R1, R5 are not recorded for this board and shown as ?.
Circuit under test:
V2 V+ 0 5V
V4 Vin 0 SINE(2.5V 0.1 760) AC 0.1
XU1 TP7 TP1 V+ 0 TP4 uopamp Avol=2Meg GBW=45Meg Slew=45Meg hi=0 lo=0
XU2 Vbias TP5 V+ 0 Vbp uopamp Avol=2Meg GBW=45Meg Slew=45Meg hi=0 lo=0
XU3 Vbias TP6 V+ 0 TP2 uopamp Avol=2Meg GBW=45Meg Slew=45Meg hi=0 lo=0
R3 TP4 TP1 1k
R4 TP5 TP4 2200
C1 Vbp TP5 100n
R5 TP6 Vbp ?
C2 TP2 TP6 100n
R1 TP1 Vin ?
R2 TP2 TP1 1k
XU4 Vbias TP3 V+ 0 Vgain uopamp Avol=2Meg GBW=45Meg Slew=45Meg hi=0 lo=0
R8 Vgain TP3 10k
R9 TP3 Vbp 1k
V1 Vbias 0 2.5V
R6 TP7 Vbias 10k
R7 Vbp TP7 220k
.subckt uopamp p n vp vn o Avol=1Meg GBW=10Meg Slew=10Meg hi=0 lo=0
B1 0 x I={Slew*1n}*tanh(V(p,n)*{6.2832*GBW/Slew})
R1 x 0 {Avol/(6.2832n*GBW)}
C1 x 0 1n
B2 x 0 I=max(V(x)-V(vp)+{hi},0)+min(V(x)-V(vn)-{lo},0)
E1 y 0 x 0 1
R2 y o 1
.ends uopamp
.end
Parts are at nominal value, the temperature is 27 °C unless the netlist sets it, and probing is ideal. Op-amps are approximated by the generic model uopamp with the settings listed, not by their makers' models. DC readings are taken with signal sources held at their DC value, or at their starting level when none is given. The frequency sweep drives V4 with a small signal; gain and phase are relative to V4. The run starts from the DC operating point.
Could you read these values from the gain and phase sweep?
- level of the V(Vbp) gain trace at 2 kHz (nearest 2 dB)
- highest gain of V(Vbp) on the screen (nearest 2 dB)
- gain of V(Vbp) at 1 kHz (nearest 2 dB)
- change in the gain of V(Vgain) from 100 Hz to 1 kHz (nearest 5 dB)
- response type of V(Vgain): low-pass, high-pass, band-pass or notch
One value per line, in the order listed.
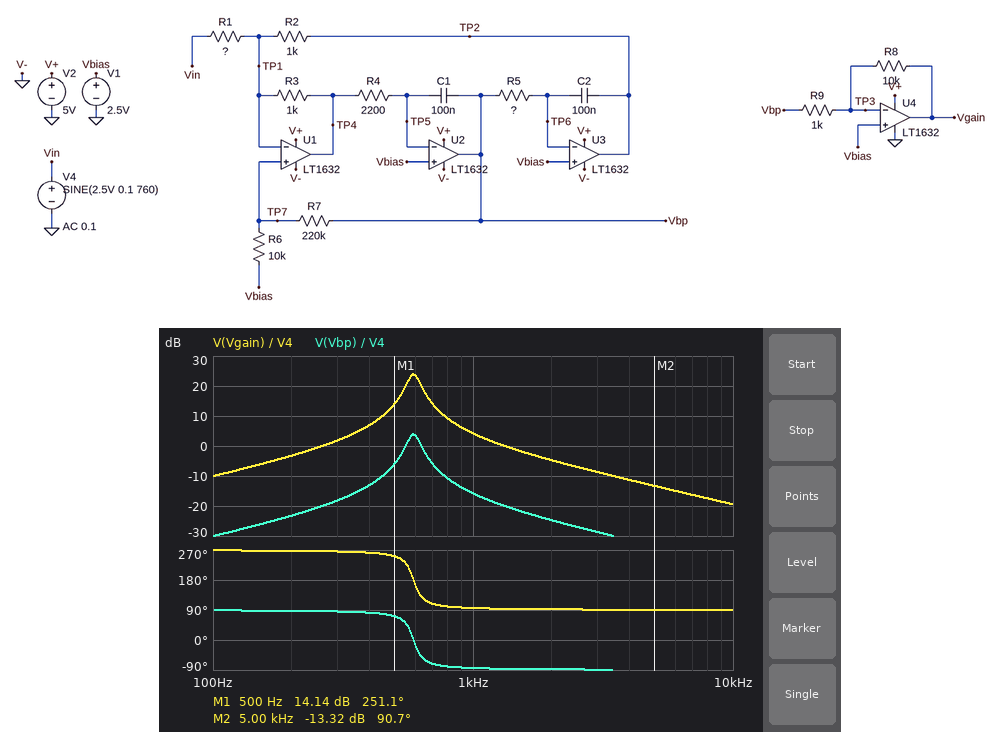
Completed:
-24 dB
4 dB
-16 dB
15 dB
band-pass
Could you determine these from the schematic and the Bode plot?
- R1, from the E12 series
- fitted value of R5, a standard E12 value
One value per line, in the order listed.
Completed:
6.8 kΩ
3.3 kΩ
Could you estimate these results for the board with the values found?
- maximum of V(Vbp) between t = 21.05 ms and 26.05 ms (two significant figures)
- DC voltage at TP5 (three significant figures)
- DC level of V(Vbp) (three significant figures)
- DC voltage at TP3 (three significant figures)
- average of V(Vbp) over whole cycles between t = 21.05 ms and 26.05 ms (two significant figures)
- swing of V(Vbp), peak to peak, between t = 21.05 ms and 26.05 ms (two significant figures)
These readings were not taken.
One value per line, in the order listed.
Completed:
2.5 V
2.50 V
2.50 V
2.50 V
2.5 V
69 mV
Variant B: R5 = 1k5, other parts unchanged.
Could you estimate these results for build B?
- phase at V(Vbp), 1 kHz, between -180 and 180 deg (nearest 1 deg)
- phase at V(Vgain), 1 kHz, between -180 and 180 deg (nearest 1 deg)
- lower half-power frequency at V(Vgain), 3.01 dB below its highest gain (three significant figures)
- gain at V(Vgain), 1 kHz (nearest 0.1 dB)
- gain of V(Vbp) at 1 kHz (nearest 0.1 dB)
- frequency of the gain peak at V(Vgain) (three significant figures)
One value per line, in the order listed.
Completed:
-74 deg
106 deg
843 Hz
12.9 dB
-7.1 dB
876 Hz
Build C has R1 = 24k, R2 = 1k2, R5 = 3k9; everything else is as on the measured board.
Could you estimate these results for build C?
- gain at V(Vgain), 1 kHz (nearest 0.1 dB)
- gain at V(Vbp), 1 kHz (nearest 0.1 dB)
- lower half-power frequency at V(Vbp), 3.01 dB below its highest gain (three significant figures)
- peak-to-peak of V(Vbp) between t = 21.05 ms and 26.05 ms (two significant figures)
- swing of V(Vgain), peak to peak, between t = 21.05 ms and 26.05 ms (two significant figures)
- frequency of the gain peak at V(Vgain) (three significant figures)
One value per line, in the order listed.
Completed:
-8.0 dB
-28.0 dB
467 Hz
14 mV
140 mV
496 Hz
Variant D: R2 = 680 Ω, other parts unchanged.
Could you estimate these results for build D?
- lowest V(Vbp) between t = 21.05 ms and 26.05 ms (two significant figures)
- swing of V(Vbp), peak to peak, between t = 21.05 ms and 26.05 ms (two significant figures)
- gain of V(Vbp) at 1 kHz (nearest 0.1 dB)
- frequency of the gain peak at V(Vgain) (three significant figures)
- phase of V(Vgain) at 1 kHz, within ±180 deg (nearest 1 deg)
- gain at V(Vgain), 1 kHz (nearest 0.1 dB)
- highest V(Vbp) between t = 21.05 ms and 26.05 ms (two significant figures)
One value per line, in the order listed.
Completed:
2.4 V
180 mV
-13.3 dB
716 Hz
100 deg
6.7 dB
2.6 V
